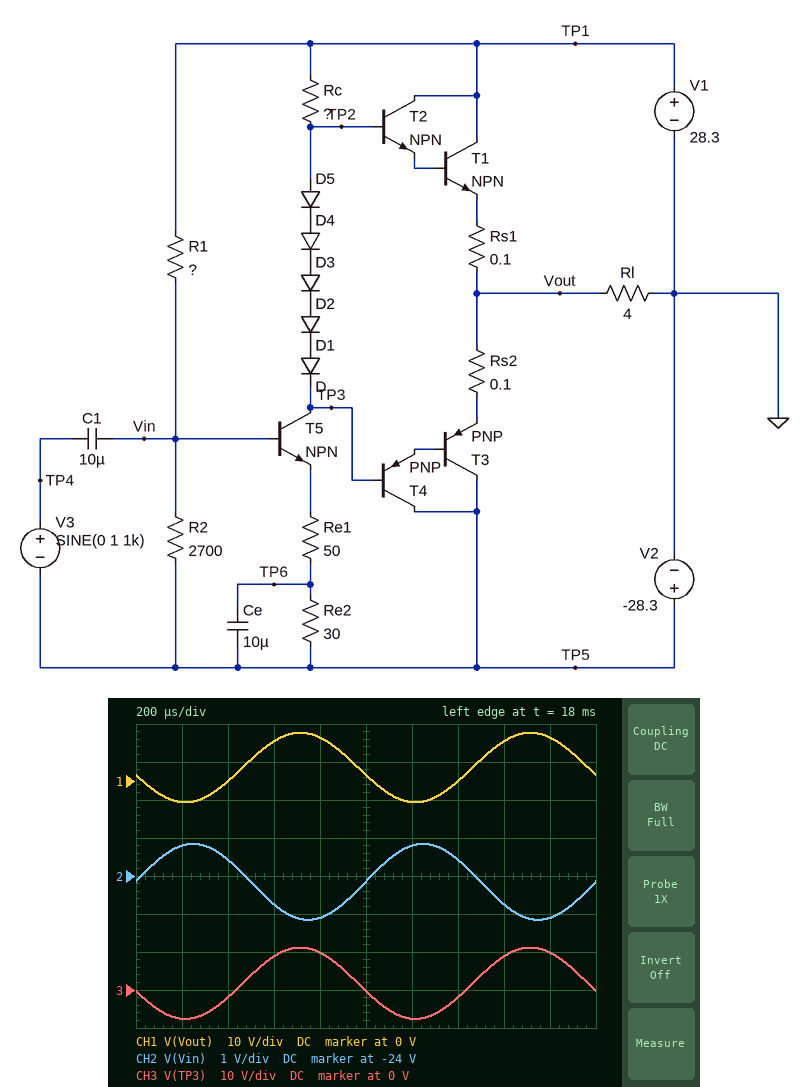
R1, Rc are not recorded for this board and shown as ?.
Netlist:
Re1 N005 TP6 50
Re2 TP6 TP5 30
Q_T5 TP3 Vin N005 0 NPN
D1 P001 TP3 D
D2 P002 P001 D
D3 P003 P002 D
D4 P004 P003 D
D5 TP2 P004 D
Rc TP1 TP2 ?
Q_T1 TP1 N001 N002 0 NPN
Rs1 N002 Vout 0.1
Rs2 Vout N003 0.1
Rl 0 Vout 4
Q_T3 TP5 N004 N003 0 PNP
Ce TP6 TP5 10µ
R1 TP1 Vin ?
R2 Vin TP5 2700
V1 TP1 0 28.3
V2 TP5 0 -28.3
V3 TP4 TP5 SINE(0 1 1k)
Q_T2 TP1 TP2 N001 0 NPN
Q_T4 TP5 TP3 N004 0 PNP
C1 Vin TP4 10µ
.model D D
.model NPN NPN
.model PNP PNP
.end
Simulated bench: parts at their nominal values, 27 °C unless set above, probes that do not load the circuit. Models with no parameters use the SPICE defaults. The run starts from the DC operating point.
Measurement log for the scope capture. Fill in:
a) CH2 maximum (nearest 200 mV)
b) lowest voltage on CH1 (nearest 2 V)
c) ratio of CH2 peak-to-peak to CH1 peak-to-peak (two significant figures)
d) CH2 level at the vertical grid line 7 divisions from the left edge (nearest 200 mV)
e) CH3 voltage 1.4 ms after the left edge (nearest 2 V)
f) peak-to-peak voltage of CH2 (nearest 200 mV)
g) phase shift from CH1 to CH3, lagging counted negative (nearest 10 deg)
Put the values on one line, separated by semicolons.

-23.2 V; -6 V; 0.11; -23.6 V; -2 V; 2.0 V; 0 deg
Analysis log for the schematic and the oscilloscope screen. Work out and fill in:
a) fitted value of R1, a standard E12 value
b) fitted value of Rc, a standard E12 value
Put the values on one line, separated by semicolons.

27 kΩ; 560 Ω
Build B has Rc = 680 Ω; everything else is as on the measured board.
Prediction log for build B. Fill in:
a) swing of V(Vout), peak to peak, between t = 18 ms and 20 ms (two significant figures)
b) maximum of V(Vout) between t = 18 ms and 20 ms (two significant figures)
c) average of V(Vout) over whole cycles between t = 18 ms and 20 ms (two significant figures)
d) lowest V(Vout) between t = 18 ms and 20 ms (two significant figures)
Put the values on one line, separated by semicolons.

22 V; 9.9 V; -1.1 V; -12 V
